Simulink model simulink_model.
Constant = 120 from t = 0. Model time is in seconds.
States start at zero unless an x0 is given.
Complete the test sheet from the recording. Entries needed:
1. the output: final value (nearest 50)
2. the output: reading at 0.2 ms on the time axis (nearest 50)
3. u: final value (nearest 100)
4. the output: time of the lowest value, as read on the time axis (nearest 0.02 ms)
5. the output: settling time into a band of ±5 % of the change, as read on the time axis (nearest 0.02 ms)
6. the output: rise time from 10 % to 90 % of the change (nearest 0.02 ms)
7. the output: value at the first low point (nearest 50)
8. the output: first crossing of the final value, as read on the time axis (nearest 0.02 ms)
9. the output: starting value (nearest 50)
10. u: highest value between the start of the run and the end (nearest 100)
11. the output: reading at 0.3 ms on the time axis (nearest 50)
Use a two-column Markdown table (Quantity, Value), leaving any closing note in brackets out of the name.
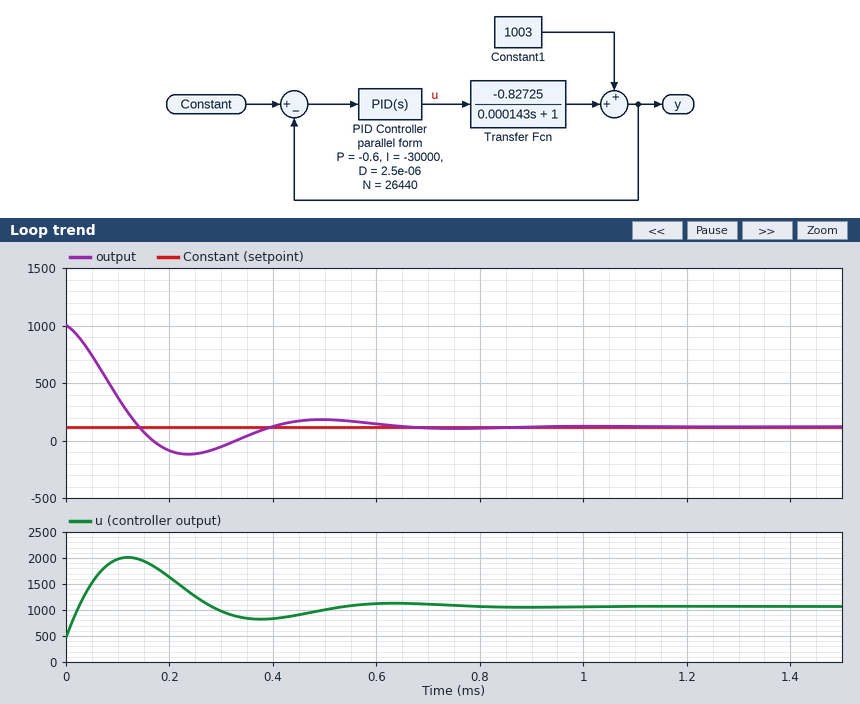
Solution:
| Quantity | Value |
|---|---|
| the output: final value | 100 |
| the output: reading at 0.2 ms on the time axis | -100 |
| u: final value | 1100 |
| the output: time of the lowest value, as read on the time axis | 0.24 ms |
| the output: settling time into a band of ±5 % of the change, as read on the time axis | 0.56 ms |
| the output: rise time from 10 % to 90 % of the change | 0.10 ms |
| the output: value at the first low point | -100 |
| the output: first crossing of the final value, as read on the time axis | 0.14 ms |
| the output: starting value | 1000 |
| u: highest value between the start of the run and the end | 2000 |
| the output: reading at 0.3 ms on the time axis | -50 |
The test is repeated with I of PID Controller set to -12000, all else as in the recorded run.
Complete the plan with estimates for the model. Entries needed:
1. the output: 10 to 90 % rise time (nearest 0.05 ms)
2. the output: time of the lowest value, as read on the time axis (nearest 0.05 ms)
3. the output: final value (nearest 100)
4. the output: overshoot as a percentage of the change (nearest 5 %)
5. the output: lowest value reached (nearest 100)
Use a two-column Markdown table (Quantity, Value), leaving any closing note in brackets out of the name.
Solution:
| Quantity | Value |
|---|---|
| the output: 10 to 90 % rise time | 0.20 ms |
| the output: time of the lowest value, as read on the time axis | 0.40 ms |
| the output: final value | 100 |
| the output: overshoot as a percentage of the change | 10 % |
| the output: lowest value reached | 0 |
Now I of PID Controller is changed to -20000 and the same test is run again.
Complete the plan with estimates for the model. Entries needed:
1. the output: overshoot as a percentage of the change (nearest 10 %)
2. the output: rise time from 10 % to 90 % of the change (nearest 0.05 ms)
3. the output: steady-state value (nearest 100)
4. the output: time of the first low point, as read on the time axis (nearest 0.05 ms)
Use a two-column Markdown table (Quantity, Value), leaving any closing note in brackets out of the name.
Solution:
| Quantity | Value |
|---|---|
| the output: overshoot as a percentage of the change | 20 % |
| the output: rise time from 10 % to 90 % of the change | 0.15 ms |
| the output: steady-state value | 100 |
| the output: time of the first low point, as read on the time axis | 0.30 ms |
